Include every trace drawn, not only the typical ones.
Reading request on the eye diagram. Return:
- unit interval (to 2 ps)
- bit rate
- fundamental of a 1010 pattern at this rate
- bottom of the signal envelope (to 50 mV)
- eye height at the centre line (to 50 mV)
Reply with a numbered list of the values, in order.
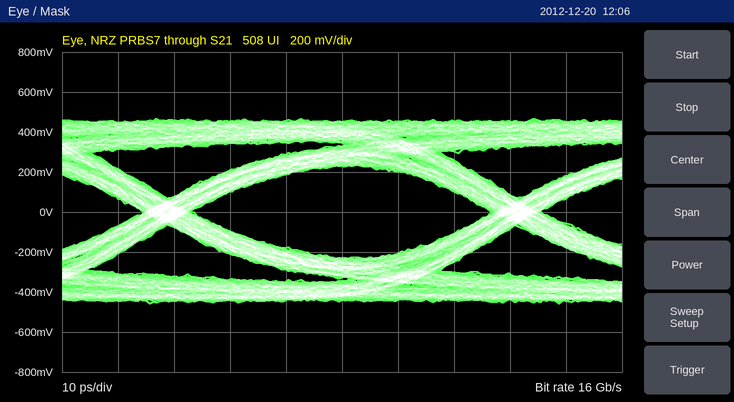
1. 62 ps
2. 16 Gb/s
3. 8 GHz
4. -450 mV
5. 450 mV
